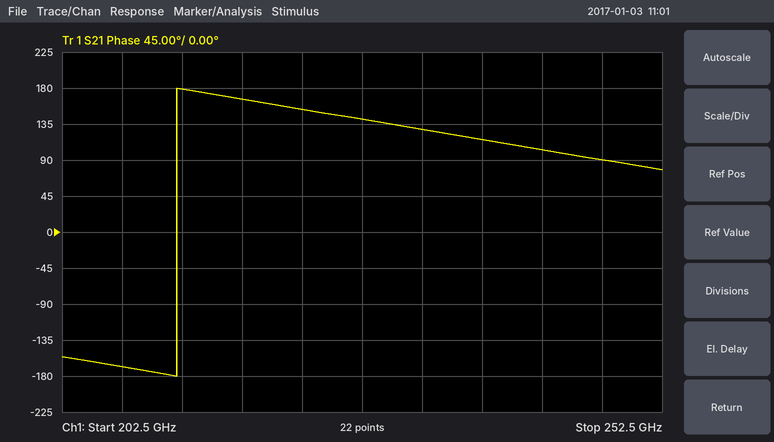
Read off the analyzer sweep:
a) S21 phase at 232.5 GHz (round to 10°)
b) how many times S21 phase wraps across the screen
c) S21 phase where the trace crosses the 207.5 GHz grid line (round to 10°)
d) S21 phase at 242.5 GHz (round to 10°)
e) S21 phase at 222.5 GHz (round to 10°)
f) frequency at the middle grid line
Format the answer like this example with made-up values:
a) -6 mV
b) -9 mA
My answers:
a) 130°
b) 1
c) -170°
d) 100°
e) 150°
f) 227.5 GHz
